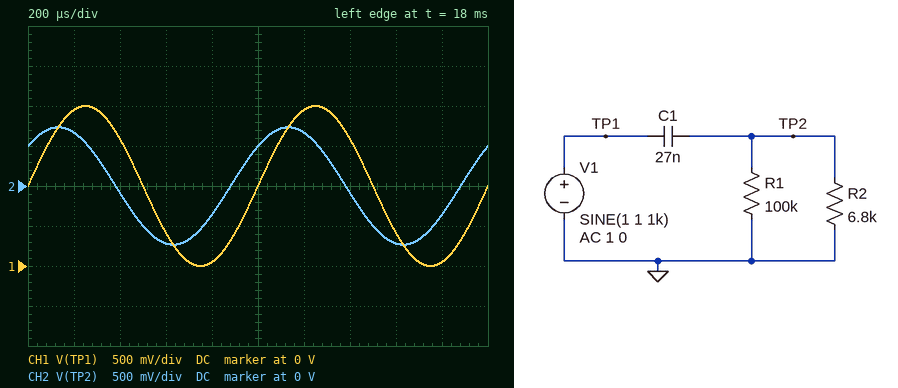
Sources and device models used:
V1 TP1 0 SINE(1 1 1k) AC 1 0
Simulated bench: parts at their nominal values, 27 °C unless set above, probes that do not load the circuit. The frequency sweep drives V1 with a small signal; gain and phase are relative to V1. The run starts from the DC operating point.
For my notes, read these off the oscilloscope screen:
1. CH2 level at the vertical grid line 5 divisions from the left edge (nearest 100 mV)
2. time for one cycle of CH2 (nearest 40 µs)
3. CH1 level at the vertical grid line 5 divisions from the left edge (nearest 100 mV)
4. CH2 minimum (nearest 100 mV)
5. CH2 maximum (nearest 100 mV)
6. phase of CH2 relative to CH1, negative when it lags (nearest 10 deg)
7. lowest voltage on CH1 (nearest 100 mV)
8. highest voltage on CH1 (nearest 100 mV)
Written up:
500 mV
1.00 ms
1.0 V
-700 mV
700 mV
40 deg
0 V
2.0 V
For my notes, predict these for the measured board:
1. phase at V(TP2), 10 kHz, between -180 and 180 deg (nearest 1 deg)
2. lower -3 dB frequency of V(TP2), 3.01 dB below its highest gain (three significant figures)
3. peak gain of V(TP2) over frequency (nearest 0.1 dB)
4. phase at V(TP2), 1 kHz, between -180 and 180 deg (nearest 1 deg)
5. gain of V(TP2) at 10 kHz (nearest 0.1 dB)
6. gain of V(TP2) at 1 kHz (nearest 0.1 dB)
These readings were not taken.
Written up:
5 deg
926 Hz
0 dB
43 deg
0 dB
-2.7 dB
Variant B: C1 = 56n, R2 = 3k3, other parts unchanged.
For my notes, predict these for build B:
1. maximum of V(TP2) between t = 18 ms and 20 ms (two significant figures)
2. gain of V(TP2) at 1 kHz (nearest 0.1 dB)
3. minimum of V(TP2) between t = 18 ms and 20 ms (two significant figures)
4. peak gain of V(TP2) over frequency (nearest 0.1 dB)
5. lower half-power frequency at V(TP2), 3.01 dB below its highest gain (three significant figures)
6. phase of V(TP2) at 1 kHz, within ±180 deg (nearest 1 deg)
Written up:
750 mV
-2.5 dB
-750 mV
0 dB
890 Hz
42 deg
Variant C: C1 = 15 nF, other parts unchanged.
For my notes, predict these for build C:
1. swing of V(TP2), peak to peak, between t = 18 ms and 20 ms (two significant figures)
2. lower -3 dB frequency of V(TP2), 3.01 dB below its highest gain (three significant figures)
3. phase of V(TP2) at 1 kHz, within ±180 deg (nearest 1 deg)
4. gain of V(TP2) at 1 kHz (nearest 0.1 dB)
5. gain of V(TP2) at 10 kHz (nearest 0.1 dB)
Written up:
1.0 V
1.67 kHz
59 deg
-5.8 dB
-0.1 dB
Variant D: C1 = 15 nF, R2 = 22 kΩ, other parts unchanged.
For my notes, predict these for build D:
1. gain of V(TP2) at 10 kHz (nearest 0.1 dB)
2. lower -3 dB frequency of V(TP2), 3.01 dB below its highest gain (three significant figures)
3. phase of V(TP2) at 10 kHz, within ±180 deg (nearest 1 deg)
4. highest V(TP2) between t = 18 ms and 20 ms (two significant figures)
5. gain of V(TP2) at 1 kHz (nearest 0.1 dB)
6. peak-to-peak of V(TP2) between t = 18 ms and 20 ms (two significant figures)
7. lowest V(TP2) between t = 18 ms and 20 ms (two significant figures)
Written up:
0 dB
588 Hz
3 deg
860 mV
-1.3 dB
1.7 V
-860 mV
